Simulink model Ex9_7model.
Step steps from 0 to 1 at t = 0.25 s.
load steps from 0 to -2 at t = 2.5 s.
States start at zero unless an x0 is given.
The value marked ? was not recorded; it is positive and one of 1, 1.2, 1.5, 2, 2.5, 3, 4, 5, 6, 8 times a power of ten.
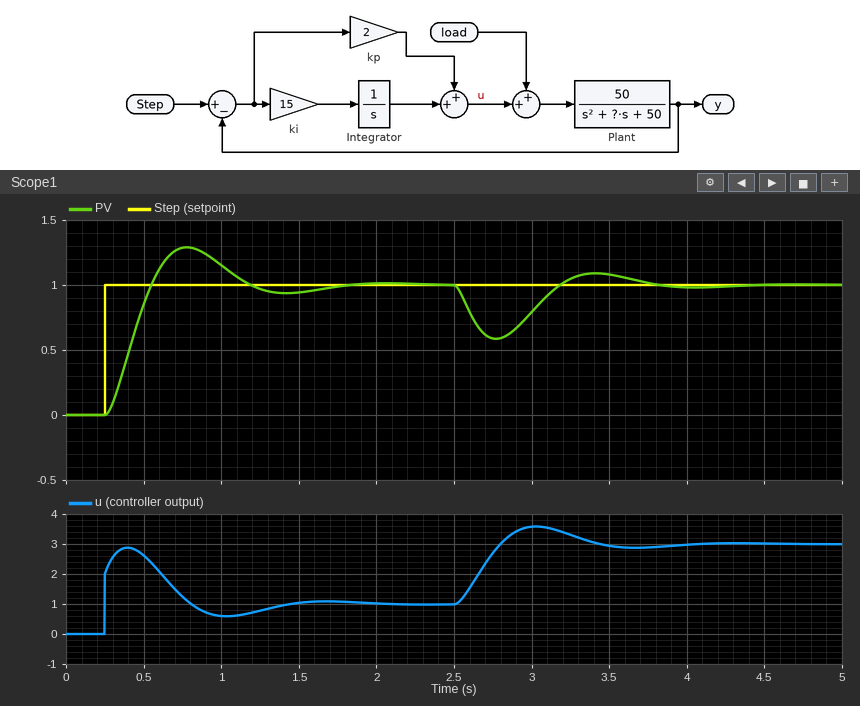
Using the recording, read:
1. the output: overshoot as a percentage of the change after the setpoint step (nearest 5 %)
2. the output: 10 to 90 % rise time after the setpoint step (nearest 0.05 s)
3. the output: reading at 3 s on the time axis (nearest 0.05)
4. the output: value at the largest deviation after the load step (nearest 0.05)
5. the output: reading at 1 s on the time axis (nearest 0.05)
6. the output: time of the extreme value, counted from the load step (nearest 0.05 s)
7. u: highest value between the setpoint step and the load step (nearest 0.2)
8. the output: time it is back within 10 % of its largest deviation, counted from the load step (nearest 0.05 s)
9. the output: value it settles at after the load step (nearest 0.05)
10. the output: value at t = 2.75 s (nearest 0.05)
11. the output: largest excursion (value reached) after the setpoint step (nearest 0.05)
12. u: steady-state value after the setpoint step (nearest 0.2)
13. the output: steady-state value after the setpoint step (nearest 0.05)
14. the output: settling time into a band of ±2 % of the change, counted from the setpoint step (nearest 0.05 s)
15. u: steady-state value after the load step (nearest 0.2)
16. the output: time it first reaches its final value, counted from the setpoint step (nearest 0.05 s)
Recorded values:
30 %
0.20 s
0.80
0.60
1.15
0.25 s
2.8
1.15 s
1.00
0.60
1.30
1.0
1.00
1.45 s
3.0
0.30 s
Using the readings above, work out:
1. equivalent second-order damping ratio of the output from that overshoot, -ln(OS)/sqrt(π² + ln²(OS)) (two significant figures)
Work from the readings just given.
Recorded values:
0.36
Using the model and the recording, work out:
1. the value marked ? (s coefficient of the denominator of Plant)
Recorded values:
30
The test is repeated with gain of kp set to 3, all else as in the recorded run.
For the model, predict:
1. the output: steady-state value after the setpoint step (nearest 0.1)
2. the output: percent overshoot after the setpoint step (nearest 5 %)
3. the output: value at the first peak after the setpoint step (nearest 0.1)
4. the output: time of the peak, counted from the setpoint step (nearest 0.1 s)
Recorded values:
1.0
20 %
1.2
0.5 s
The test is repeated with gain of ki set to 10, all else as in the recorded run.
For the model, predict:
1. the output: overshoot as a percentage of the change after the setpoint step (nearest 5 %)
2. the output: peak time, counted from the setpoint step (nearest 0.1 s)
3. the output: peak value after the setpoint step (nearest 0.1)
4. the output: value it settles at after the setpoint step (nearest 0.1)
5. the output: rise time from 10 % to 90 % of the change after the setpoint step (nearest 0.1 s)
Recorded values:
20 %
0.6 s
1.2
1.0
0.3 s
